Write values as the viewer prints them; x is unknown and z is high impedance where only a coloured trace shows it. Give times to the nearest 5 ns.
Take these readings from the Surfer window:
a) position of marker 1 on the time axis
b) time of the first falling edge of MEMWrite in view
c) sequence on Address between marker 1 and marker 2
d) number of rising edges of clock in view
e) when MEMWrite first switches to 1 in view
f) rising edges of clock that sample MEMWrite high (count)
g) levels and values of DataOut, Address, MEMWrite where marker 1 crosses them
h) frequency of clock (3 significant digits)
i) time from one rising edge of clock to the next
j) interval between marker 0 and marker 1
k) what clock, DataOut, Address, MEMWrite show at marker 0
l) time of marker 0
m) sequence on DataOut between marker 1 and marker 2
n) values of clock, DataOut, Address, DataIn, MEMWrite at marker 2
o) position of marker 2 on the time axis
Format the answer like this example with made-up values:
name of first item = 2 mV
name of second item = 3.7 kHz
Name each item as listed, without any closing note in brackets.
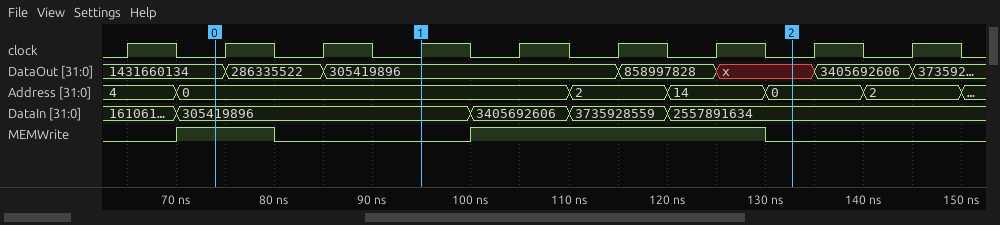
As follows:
position of marker 1 on the time axis = 95 ns
time of the first falling edge of MEMWrite in view = 80 ns
sequence on Address between marker 1 and marker 2 = 0, 2, 14, 0
number of rising edges of clock in view = 9
when MEMWrite first switches to 1 in view = 70 ns
rising edges of clock that sample MEMWrite high = 4
levels and values of DataOut, Address, MEMWrite where marker 1 crosses them = DataOut=305419896, Address=0, MEMWrite=0
frequency of clock = 100 MHz
time from one rising edge of clock to the next = 10 ns
interval between marker 0 and marker 1 = 20 ns
what clock, DataOut, Address, MEMWrite show at marker 0 = clock=0, DataOut=1431660134, Address=0, MEMWrite=1
time of marker 0 = 75 ns
sequence on DataOut between marker 1 and marker 2 = 305419896, 858997828, x
values of clock, DataOut, Address, DataIn, MEMWrite at marker 2 = clock=0, DataOut=x, Address=0, DataIn=2557891634, MEMWrite=0
position of marker 2 on the time axis = 135 ns
